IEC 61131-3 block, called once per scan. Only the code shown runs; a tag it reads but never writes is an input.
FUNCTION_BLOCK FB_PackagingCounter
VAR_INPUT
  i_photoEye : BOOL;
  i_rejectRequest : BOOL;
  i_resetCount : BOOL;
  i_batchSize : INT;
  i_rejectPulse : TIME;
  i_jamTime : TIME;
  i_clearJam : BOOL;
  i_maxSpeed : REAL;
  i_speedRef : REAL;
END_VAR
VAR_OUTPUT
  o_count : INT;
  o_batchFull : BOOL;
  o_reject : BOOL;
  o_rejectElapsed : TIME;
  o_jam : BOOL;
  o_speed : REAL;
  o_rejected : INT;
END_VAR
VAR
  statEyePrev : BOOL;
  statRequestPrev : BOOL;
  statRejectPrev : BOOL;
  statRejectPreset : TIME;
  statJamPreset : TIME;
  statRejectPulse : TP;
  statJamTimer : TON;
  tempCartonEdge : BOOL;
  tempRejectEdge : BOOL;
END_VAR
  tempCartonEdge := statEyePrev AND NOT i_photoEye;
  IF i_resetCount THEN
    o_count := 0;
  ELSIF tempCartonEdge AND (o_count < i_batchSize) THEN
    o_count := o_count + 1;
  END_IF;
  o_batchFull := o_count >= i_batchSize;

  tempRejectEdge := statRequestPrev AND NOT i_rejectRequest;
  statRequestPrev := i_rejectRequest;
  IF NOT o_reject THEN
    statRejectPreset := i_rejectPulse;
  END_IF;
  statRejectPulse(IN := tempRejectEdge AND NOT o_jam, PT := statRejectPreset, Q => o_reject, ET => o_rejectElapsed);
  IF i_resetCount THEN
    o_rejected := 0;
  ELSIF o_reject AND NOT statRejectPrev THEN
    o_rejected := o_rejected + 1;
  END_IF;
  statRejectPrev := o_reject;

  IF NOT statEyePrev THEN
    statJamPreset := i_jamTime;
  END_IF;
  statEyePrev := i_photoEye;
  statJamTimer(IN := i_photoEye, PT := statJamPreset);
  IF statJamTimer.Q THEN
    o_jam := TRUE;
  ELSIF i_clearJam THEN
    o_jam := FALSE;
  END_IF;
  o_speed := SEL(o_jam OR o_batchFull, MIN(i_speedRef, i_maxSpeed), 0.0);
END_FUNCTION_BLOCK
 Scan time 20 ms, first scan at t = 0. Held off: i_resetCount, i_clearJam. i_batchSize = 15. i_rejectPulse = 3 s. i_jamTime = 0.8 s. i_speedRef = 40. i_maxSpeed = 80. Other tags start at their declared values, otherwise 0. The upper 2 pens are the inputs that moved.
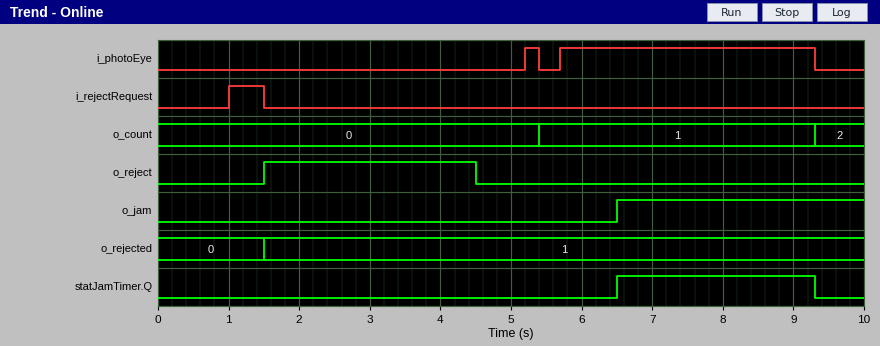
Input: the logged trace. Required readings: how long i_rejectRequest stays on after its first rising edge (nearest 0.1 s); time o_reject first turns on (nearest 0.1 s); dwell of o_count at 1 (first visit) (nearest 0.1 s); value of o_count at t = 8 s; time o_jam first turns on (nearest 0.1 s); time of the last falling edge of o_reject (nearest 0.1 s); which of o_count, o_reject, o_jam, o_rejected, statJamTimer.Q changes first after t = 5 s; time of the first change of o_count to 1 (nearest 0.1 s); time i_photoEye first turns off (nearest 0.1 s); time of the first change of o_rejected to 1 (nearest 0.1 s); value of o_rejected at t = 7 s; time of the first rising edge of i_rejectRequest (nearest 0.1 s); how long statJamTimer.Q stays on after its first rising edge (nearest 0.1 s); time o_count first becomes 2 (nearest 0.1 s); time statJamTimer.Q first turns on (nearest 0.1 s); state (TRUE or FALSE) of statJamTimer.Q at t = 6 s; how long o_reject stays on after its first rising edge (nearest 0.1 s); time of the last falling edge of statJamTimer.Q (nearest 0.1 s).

0.5 s
1.5 s
3.9 s
1
6.5 s
4.5 s
o_count
5.4 s
5.4 s
1.5 s
1
1.0 s
2.8 s
9.3 s
6.5 s
FALSE
3.0 s
9.3 s
